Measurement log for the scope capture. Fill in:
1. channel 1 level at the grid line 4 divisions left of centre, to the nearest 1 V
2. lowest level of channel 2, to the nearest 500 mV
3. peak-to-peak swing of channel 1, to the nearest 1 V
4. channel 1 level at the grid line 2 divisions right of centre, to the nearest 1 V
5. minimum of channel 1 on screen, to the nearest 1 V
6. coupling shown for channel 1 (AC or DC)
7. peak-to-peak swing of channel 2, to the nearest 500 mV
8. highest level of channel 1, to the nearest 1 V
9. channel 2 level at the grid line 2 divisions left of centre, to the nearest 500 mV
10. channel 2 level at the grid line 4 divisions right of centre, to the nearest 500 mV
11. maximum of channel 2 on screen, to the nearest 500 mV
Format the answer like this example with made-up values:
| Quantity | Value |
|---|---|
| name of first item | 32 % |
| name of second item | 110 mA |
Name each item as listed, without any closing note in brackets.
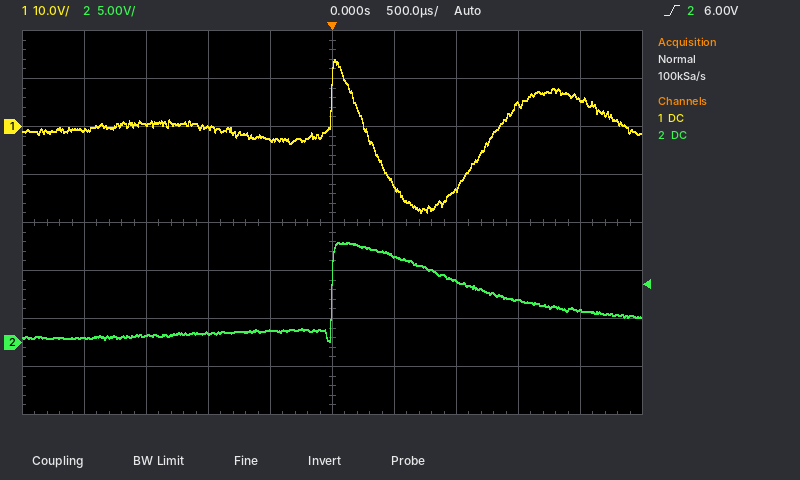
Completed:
| Quantity | Value |
|---|---|
| channel 1 level at the grid line 4 divisions left of centre, to the nearest 1 V | -1 V |
| lowest level of channel 2, to the nearest 500 mV | 0.0 V |
| peak-to-peak swing of channel 1, to the nearest 1 V | 32 V |
| channel 1 level at the grid line 2 divisions right of centre, to the nearest 1 V | -13 V |
| minimum of channel 1 on screen, to the nearest 1 V | -18 V |
| coupling shown for channel 1 | DC |
| peak-to-peak swing of channel 2, to the nearest 500 mV | 10.5 V |
| highest level of channel 1, to the nearest 1 V | 14 V |
| channel 2 level at the grid line 2 divisions left of centre, to the nearest 500 mV | 1.0 V |
| channel 2 level at the grid line 4 divisions right of centre, to the nearest 500 mV | 3.5 V |
| maximum of channel 2 on screen, to the nearest 500 mV | 10.5 V |
